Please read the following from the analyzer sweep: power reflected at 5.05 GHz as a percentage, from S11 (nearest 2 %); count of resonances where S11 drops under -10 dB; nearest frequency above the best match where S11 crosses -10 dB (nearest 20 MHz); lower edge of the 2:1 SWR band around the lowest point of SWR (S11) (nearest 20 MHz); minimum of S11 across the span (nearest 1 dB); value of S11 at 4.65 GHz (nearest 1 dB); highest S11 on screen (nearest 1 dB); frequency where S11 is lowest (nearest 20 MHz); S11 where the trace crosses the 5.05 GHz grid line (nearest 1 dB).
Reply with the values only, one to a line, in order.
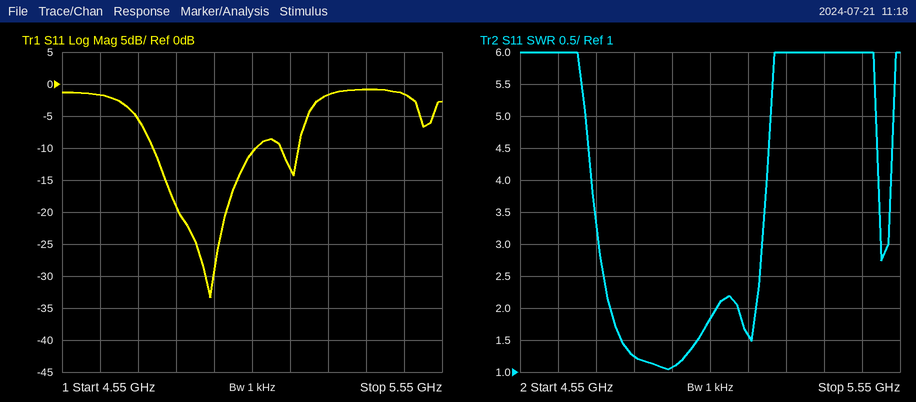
8 %
2
5.06 GHz
4.78 GHz
-33 dB
-2 dB
-1 dB
4.94 GHz
-11 dB
